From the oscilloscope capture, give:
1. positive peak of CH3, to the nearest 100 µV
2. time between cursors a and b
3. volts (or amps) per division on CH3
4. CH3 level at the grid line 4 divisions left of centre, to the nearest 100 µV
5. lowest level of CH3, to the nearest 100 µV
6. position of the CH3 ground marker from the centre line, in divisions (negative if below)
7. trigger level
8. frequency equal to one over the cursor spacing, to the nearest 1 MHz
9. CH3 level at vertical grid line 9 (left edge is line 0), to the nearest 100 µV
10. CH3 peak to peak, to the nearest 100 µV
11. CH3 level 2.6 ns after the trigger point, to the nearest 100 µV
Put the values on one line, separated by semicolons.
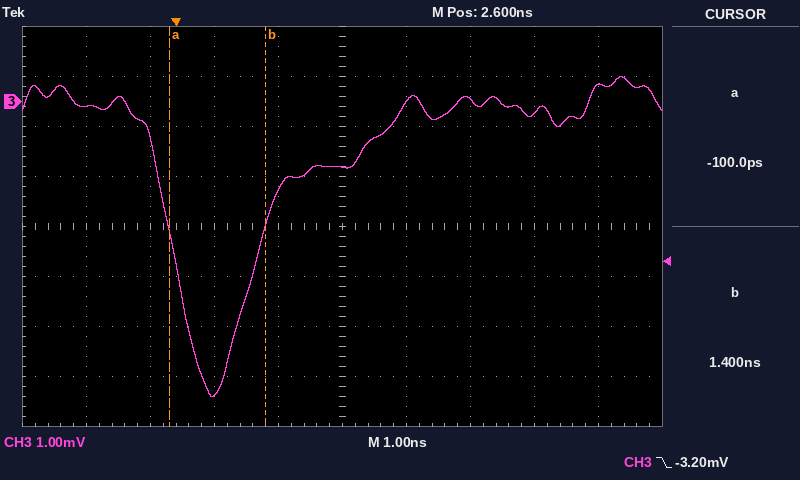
500 µV; 1.5 ns; 1 mV; -100 µV; -5.9 mV; +2.5 div; -3.20 mV; 667 MHz; 300 µV; 6.4 mV; -1.3 mV
